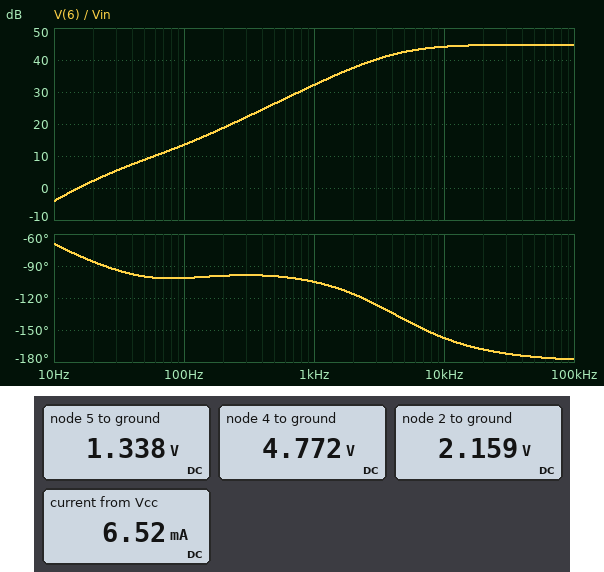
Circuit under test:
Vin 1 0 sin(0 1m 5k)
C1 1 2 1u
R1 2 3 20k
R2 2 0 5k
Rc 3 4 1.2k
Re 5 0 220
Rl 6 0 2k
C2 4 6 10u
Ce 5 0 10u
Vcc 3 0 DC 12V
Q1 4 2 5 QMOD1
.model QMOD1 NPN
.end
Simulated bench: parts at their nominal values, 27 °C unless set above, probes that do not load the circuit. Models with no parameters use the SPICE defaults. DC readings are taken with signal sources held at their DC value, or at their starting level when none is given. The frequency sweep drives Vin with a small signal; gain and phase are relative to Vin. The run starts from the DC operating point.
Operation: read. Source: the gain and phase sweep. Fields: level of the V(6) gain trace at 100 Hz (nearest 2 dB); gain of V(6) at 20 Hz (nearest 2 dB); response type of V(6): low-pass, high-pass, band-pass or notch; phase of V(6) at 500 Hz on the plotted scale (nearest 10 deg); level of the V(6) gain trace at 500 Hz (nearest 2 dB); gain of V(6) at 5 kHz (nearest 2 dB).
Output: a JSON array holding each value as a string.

["14 dB", "2 dB", "high-pass", "-100 deg", "26 dB", "42 dB"]
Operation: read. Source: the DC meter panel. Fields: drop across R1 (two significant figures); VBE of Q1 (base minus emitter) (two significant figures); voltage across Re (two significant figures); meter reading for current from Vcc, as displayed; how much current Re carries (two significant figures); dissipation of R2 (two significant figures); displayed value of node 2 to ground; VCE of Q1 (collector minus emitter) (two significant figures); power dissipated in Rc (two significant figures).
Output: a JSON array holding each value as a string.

["9.8 V", "820 mV", "1.3 V", "6.52 mA", "6.1 mA", "930 µW", "2.159 V", "3.4 V", "44 mW"]
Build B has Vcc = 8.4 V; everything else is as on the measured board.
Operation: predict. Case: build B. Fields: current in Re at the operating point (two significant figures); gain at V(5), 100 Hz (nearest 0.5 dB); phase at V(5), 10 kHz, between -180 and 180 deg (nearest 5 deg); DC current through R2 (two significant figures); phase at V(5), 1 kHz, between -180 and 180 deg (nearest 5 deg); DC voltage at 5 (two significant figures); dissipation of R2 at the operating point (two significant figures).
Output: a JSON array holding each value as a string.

["3.4 mA", "-2.0 dB", "-75 deg", "310 µA", "-20 deg", "740 mV", "480 µW"]
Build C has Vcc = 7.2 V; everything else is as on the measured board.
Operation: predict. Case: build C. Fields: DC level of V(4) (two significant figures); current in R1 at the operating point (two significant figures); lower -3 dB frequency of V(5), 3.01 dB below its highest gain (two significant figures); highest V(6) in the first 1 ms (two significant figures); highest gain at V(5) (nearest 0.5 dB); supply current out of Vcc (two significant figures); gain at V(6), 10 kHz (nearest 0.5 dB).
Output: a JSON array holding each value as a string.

["4.3 V", "290 µA", "41 Hz", "71 mV", "-1.5 dB", "2.7 mA", "37.0 dB"]
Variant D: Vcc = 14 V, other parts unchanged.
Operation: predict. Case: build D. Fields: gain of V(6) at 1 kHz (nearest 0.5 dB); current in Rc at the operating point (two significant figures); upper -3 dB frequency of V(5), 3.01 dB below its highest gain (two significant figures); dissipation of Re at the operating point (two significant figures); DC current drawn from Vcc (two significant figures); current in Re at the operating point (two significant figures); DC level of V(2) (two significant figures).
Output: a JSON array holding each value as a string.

["32.5 dB", "7.5 mA", "5.3 kHz", "13 mW", "8.1 mA", "7.6 mA", "2.5 V"]
